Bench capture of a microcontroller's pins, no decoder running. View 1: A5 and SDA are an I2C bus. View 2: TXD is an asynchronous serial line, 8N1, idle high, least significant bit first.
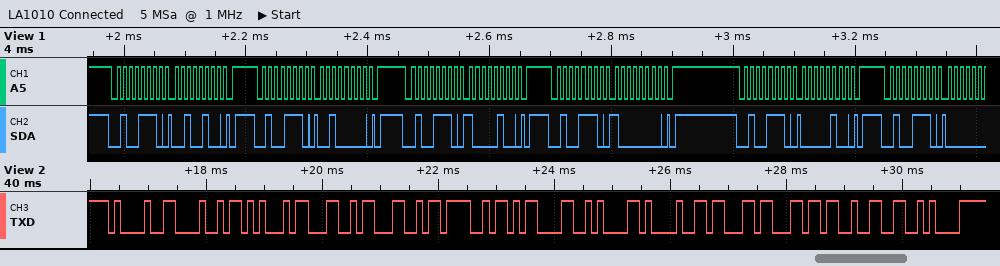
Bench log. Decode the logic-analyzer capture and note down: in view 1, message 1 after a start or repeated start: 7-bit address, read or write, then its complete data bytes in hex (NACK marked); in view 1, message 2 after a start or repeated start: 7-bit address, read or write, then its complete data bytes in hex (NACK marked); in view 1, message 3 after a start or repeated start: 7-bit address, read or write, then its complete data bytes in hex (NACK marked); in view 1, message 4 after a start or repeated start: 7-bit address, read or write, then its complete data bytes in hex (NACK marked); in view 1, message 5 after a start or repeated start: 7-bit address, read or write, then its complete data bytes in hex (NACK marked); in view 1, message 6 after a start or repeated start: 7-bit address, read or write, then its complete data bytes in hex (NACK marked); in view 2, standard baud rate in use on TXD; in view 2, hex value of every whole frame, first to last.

0x27 write: 24
0x27 write: 20
0x27 write: 84
0x27 write: 80
0x27 write: 04
0x27 write
9600 baud
21 48 45 4C 4C 4F 0D 0A 21 63 6C 32 0A
